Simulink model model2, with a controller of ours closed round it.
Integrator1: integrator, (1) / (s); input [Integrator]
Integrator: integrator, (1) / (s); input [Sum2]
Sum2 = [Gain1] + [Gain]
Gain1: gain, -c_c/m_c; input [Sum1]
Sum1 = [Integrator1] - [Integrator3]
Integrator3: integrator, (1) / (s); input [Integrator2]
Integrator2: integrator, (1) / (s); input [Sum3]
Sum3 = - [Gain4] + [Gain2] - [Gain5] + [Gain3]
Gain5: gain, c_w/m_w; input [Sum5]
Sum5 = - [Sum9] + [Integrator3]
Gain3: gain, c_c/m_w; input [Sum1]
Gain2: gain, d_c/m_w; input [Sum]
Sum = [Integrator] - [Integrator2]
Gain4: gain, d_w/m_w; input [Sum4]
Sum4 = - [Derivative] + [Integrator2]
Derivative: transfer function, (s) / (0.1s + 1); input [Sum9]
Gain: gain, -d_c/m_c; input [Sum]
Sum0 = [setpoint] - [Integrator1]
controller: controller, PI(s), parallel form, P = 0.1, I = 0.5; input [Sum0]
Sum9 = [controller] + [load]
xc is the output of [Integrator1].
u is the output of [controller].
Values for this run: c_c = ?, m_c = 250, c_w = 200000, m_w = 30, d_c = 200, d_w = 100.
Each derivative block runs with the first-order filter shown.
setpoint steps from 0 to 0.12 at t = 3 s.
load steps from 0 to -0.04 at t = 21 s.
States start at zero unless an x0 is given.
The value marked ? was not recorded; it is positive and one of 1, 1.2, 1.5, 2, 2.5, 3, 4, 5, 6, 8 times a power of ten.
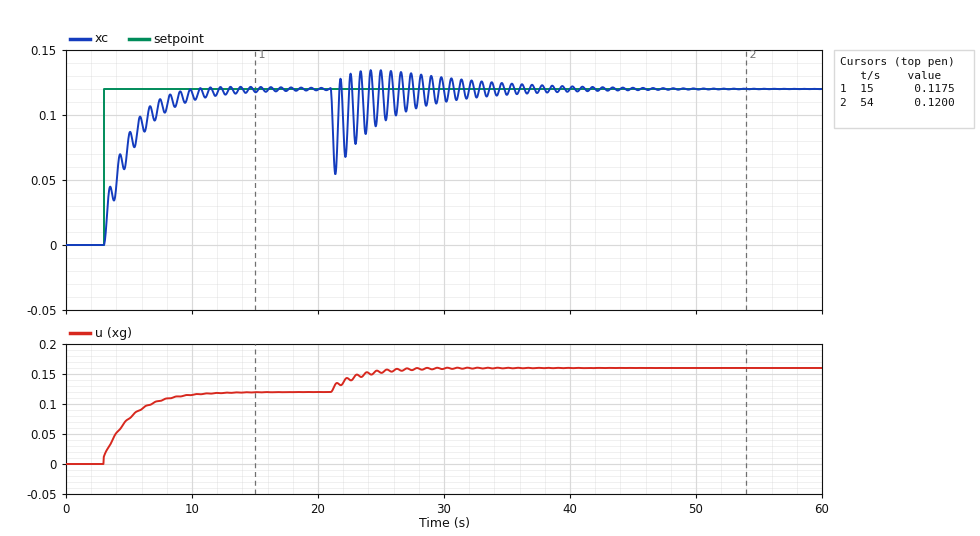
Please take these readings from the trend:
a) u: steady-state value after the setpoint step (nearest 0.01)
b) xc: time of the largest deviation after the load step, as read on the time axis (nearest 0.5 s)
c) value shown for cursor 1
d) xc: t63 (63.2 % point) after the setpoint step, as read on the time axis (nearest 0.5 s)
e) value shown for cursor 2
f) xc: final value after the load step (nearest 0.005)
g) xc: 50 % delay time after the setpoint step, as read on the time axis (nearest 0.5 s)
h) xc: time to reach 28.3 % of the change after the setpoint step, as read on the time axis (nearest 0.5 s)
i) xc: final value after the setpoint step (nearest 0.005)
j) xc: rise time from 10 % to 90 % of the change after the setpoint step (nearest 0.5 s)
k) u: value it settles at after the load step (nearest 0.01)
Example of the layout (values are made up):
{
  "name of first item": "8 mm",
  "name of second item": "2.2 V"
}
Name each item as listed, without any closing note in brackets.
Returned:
{
  "u: steady-state value after the setpoint step": "0.12",
  "xc: time of the largest deviation after the load step, as read on the time axis": "21.5 s",
  "value shown for cursor 1": "0.1175",
  "xc: t63 (63.2 % point) after the setpoint step, as read on the time axis": "5.0 s",
  "value shown for cursor 2": "0.1200",
  "xc: final value after the load step": "0.120",
  "xc: 50 % delay time after the setpoint step, as read on the time axis": "4.0 s",
  "xc: time to reach 28.3 % of the change after the setpoint step, as read on the time axis": "3.5 s",
  "xc: final value after the setpoint step": "0.120",
  "xc: rise time from 10 % to 90 % of the change after the setpoint step": "4.0 s",
  "u: value it settles at after the load step": "0.16"
}
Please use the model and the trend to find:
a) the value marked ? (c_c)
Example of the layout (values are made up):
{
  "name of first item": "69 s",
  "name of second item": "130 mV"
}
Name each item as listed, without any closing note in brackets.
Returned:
{
  "the value marked ?": "15000"
}
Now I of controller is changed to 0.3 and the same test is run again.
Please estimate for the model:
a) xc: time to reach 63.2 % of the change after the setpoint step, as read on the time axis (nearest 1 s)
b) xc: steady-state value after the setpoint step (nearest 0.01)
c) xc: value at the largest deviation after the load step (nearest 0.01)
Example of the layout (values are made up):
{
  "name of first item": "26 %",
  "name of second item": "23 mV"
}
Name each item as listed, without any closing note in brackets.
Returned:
{
  "xc: time to reach 63.2 % of the change after the setpoint step, as read on the time axis": "6 s",
  "xc: steady-state value after the setpoint step": "0.12",
  "xc: value at the largest deviation after the load step": "0.05"
}
